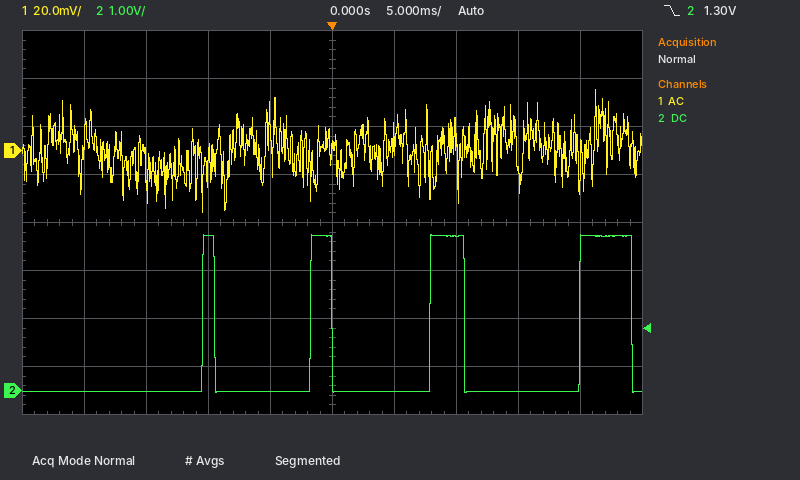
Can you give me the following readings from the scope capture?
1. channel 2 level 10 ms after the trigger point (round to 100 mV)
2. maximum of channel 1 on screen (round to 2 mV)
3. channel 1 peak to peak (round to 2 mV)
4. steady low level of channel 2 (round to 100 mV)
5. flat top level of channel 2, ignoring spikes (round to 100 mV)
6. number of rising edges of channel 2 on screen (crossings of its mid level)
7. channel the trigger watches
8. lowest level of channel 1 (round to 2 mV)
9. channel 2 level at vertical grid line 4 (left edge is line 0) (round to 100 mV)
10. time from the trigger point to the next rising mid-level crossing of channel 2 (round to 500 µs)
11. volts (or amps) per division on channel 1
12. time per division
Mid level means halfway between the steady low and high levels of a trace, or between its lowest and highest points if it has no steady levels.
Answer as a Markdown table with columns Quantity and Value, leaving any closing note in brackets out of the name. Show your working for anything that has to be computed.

| Quantity | Value |
|---|---|
| channel 2 level 10 ms after the trigger point | 3.2 V |
| maximum of channel 1 on screen | 26 mV |
| channel 1 peak to peak | 26 mV − (-26 mV) = 52 mV |
| steady low level of channel 2 | 0.0 V |
| flat top level of channel 2, ignoring spikes | 3.2 V |
| number of rising edges of channel 2 on screen | 4 |
| channel the trigger watches | channel 2 |
| lowest level of channel 1 | -26 mV |
| channel 2 level at vertical grid line 4 (left edge is line 0) | 0.0 V |
| time from the trigger point to the next rising mid-level crossing of channel 2 | 8.0 ms |
| volts (or amps) per division on channel 1 | 20 mV |
| time per division | 5 ms |
